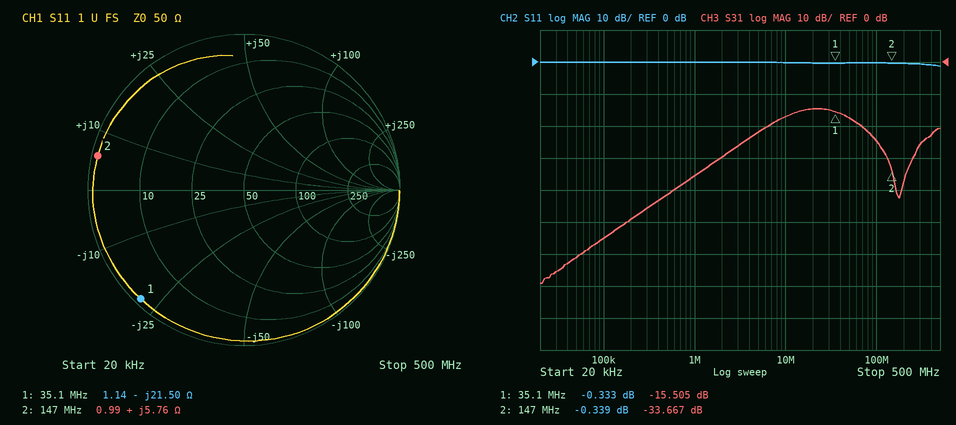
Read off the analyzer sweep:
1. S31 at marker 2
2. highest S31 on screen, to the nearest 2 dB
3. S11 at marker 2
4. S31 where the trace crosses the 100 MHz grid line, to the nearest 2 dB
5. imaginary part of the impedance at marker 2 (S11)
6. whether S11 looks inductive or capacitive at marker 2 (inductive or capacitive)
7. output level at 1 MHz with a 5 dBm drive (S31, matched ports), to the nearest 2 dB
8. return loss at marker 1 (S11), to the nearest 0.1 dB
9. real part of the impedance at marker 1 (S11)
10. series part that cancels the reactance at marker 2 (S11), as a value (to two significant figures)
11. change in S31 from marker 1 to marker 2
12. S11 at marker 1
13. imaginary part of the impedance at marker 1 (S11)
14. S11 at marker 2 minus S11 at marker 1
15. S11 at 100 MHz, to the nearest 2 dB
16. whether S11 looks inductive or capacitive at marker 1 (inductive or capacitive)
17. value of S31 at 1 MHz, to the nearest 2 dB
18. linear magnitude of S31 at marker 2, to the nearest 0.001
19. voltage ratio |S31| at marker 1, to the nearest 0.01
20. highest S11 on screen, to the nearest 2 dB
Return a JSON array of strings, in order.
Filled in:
["-33.667 dB", "-14 dB", "-0.339 dB", "-24 dB", "+5.76 Ω", "inductive", "-30 dBm", "0.3 dB", "1.14 Ω", "190 pF", "-18.162 dB", "-0.333 dB", "-21.50 Ω", "-0.006 dB", "0 dB", "capacitive", "-36 dB", "0.021", "0.17", "0 dB"]
